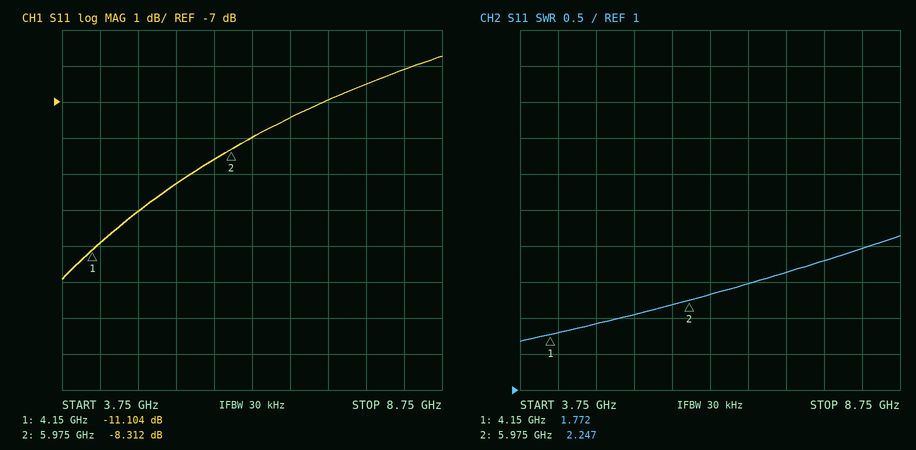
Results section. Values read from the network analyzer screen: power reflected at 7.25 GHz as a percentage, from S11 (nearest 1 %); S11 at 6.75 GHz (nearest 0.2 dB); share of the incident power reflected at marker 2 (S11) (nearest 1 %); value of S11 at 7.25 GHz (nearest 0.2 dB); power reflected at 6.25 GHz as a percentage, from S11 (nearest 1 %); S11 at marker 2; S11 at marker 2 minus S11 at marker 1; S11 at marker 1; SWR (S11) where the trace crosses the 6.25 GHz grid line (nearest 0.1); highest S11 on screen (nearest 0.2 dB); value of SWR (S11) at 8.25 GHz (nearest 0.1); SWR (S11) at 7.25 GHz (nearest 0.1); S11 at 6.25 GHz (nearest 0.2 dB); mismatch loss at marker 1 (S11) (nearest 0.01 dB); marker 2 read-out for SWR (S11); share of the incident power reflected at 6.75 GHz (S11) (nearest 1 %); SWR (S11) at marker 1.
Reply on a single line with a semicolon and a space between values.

20 %; -7.4 dB; 15 %; -7.0 dB; 16 %; -8.312 dB; 2.792 dB; -11.104 dB; 2.3; -5.8 dB; 3.0; 2.6; -8.0 dB; 0.35 dB; 2.247; 18 %; 1.772
